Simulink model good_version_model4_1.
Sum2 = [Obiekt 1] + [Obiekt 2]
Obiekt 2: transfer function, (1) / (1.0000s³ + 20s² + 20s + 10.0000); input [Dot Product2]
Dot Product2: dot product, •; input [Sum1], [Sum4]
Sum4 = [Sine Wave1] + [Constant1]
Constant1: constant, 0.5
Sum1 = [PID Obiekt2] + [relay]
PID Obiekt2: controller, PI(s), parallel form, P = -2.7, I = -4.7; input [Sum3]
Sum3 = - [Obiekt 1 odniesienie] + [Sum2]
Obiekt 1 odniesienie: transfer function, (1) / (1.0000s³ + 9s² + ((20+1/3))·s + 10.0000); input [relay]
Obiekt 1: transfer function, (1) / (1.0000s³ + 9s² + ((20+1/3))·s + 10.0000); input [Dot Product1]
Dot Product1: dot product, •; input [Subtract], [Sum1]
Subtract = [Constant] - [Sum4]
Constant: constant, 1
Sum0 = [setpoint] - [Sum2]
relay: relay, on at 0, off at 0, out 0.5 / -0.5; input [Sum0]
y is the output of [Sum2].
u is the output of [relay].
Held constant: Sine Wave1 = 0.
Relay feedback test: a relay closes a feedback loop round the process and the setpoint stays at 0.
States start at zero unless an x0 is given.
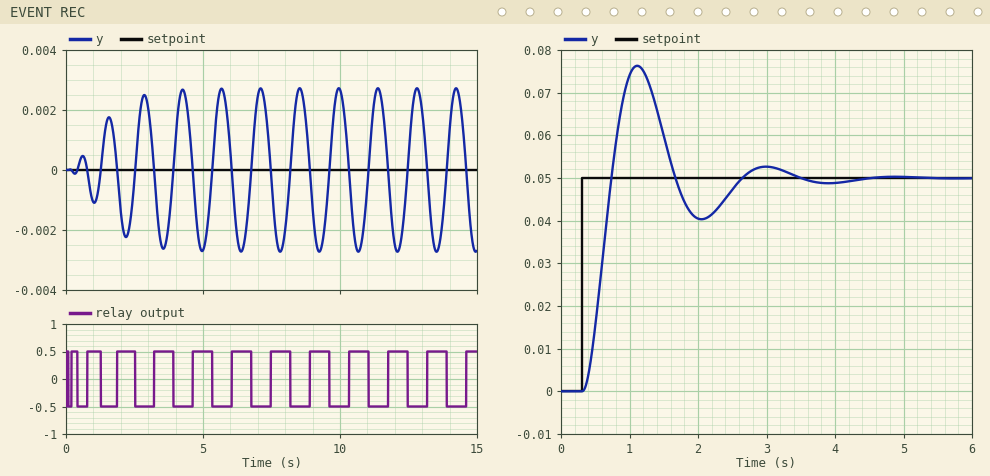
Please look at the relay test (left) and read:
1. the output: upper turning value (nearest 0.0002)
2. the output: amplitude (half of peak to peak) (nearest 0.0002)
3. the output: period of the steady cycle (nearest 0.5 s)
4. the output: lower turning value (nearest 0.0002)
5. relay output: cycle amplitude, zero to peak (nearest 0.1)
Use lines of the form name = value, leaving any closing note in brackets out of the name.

the output: upper turning value = 0.0028
the output: amplitude (half of peak to peak) = 0.0028
the output: period of the steady cycle = 1.5 s
the output: lower turning value = -0.0028
relay output: cycle amplitude, zero to peak = 0.5
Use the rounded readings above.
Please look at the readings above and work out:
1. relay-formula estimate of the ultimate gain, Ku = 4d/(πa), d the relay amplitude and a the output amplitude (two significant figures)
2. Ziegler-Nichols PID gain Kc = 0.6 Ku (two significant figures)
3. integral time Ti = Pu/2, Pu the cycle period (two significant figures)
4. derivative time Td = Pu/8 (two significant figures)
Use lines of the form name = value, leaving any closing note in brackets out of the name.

relay-formula estimate of the ultimate gain, Ku = 4d/(πa), d the relay amplitude and a the output amplitude = 230
Ziegler-Nichols PID gain Kc = 0.6 Ku = 140
integral time Ti = Pu/2, Pu the cycle period = 0.75 s
derivative time Td = Pu/8 = 0.19 s
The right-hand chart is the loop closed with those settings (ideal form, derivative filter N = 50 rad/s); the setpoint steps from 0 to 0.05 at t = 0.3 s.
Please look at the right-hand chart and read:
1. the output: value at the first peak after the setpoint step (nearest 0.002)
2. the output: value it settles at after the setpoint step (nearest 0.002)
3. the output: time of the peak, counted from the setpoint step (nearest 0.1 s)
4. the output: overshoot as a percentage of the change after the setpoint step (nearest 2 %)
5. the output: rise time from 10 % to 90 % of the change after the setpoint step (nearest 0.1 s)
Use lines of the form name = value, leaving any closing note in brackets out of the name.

the output: value at the first peak after the setpoint step = 0.076
the output: value it settles at after the setpoint step = 0.050
the output: time of the peak, counted from the setpoint step = 0.8 s
the output: overshoot as a percentage of the change after the setpoint step = 52 %
the output: rise time from 10 % to 90 % of the change after the setpoint step = 0.3 s
